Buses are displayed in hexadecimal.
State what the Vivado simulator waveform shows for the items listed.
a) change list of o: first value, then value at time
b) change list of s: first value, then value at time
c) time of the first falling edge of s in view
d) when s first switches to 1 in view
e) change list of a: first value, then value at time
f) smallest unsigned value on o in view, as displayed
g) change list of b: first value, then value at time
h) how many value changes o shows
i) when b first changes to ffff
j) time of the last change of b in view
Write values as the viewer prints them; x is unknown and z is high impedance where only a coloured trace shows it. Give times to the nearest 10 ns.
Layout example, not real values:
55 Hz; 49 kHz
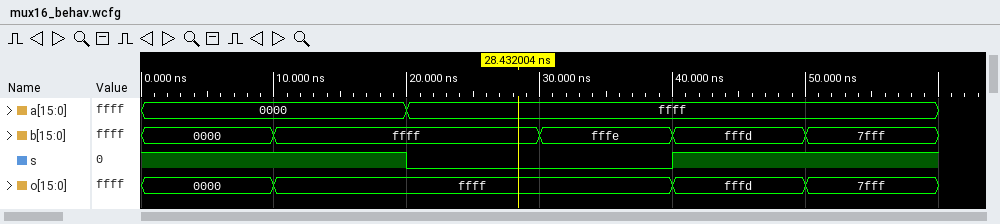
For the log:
0000, ffff at 10 ns, fffd at 40 ns, 7fff at 50 ns; 1, 0 at 20 ns, 1 at 40 ns; 20 ns; 40 ns; 0000, ffff at 20 ns; 0000; 0000, ffff at 10 ns, fffe at 30 ns, fffd at 40 ns, 7fff at 50 ns; 3; 10 ns; 50 ns
